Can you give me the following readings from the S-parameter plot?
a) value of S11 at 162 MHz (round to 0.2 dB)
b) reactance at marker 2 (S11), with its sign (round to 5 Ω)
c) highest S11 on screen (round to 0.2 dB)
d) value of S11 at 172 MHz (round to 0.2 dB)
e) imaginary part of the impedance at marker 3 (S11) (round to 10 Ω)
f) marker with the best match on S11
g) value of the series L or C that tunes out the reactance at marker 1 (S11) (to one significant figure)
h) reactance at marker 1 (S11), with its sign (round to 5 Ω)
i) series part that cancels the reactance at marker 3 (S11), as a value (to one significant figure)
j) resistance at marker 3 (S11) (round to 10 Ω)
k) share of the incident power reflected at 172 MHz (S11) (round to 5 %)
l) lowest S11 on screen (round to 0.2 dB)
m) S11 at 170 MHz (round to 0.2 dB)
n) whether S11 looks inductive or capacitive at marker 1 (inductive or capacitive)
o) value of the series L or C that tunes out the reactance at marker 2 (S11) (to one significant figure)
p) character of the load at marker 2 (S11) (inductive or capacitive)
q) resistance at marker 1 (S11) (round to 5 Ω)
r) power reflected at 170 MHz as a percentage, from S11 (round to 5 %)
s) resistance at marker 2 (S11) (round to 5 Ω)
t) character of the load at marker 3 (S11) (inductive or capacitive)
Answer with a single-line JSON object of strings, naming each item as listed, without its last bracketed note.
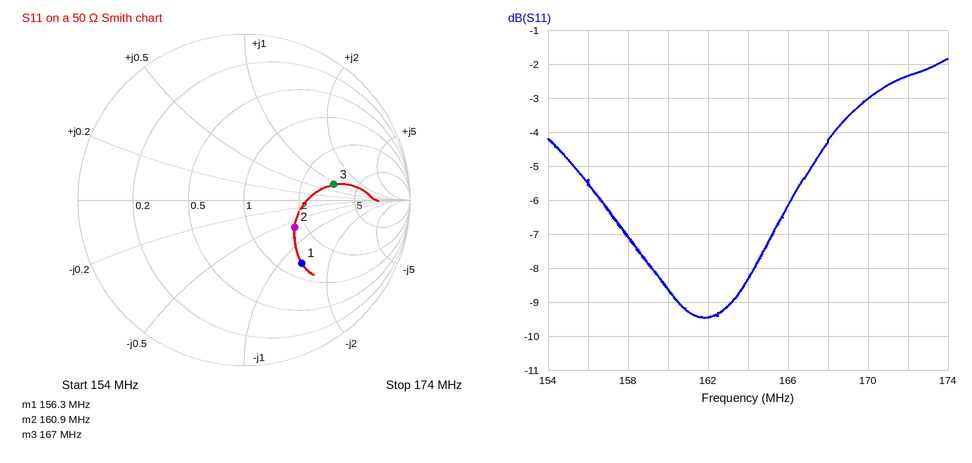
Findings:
{"value of S11 at 162 MHz": "-9.4 dB", "reactance at marker 2 (S11), with its sign": "-30 Ω", "highest S11 on screen": "-1.8 dB", "value of S11 at 172 MHz": "-2.4 dB", "imaginary part of the impedance at marker 3 (S11)": "+40 Ω", "marker with the best match on S11": "marker 2", "value of the series L or C that tunes out the reactance at marker 1 (S11)": "70 nH", "reactance at marker 1 (S11), with its sign": "-65 Ω", "series part that cancels the reactance at marker 3 (S11), as a value": "20 pF", "resistance at marker 3 (S11)": "160 Ω", "share of the incident power reflected at 172 MHz (S11)": "60 %", "lowest S11 on screen": "-9.4 dB", "S11 at 170 MHz": "-3.0 dB", "whether S11 looks inductive or capacitive at marker 1": "capacitive", "value of the series L or C that tunes out the reactance at marker 2 (S11)": "30 nH", "character of the load at marker 2 (S11)": "capacitive", "resistance at marker 1 (S11)": "65 Ω", "power reflected at 170 MHz as a percentage, from S11": "50 %", "resistance at marker 2 (S11)": "85 Ω", "character of the load at marker 3 (S11)": "inductive"}
